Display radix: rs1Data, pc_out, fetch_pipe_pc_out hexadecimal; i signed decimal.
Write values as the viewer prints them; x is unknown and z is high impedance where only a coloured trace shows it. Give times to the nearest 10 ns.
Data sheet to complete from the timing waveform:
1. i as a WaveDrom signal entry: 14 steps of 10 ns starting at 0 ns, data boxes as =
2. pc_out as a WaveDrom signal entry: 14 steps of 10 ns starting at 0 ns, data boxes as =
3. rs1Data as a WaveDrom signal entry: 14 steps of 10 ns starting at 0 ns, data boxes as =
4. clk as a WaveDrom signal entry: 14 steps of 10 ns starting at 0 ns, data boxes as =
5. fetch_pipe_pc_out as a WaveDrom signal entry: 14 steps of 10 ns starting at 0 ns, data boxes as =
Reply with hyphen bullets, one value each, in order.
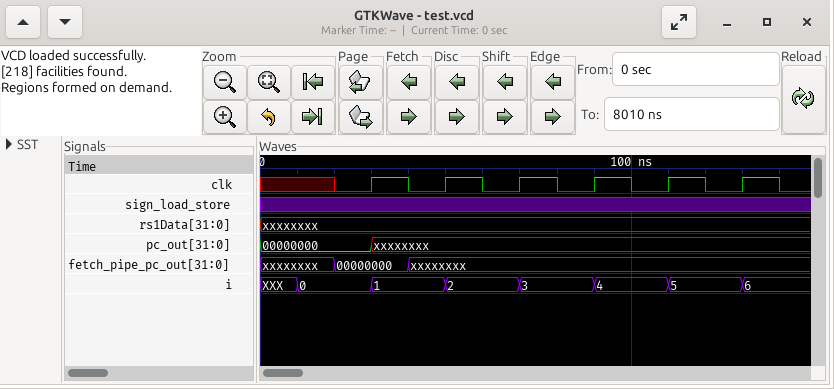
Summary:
- {name: 'i', wave: 'x=.=.=.=.=.=.=', data: '0 1 2 3 4 5 6'}
- {name: 'pc_out', wave: '=..x..........', data: '00000000'}
- {name: 'rs1Data', wave: 'x.............'}
- {name: 'clk', wave: 'x.010101010101'}
- {name: 'fetch_pipe_pc_out', wave: 'x.=.x.........', data: '00000000'}
